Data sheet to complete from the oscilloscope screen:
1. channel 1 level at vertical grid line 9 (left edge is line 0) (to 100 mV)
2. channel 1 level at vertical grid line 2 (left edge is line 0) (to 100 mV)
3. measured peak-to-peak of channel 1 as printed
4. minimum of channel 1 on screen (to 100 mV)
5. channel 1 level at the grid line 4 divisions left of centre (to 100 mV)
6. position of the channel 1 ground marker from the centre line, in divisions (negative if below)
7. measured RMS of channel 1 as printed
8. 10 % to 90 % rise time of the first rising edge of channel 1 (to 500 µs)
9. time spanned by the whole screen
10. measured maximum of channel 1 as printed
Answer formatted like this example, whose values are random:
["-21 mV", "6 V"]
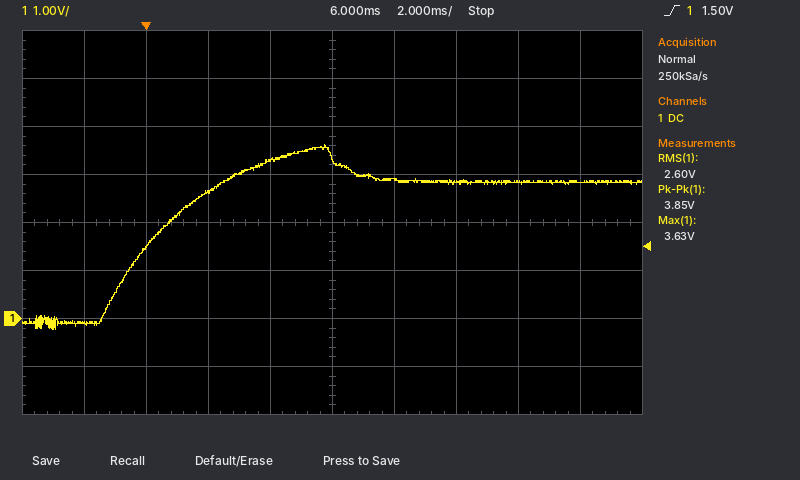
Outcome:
["2.8 V", "1.5 V", "3.85 V", "-200 mV", "-100 mV", "-2.0 div", "2.60 V", "3.0 ms", "20 ms", "3.63 V"]
